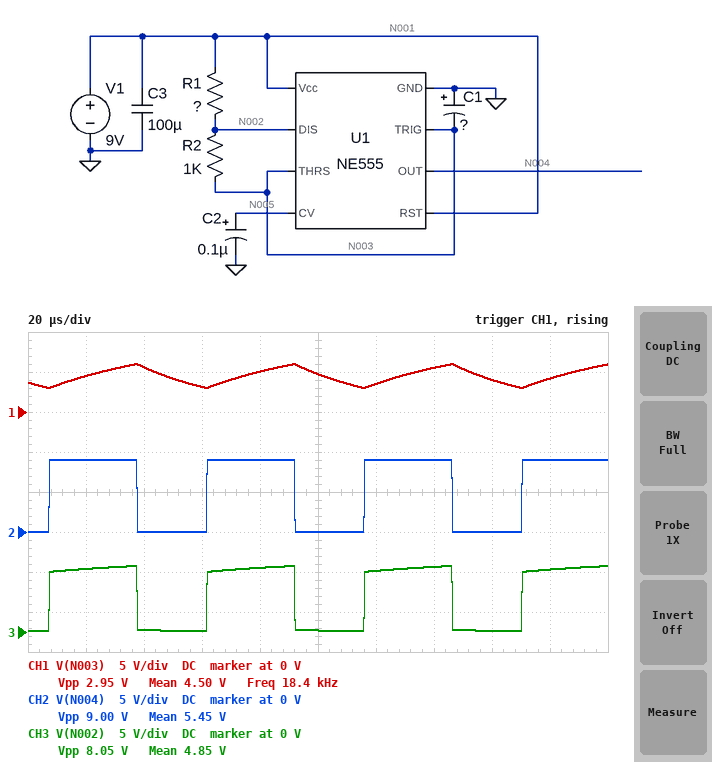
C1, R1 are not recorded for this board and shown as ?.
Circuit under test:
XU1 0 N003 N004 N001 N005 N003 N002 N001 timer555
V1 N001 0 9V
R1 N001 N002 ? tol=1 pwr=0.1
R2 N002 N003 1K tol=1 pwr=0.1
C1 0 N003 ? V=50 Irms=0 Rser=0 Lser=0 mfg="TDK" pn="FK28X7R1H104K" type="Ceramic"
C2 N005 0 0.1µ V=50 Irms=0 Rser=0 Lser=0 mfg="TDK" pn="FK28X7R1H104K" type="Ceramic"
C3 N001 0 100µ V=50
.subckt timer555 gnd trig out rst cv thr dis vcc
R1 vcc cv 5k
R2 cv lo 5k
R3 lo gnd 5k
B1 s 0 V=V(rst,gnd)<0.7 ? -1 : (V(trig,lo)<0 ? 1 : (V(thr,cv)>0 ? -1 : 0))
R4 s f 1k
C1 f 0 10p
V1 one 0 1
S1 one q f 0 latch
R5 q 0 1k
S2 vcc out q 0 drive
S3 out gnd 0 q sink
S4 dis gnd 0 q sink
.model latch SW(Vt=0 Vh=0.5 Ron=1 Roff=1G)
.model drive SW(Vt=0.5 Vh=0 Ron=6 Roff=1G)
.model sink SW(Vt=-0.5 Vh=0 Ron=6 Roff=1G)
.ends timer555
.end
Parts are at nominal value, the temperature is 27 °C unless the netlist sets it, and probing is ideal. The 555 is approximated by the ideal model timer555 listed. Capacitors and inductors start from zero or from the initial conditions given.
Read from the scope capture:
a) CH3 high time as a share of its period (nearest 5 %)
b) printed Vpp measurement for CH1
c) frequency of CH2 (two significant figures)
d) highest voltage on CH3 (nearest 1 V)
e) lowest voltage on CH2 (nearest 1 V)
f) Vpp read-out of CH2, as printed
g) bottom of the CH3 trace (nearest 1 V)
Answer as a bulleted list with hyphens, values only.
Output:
- 55 %
- 2.95 V
- 18 kHz
- 8 V
- 0 V
- 9.00 V
- 0 V
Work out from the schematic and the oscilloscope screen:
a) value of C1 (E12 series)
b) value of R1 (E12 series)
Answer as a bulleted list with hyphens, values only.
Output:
- 33 nF
- 330 Ω
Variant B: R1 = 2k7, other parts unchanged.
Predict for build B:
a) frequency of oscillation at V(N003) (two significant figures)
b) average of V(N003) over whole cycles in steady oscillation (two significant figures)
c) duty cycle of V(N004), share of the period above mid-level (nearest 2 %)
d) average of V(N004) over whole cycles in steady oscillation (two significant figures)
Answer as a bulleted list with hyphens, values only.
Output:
- 9.3 kHz
- 4.6 V
- 78 %
- 7.1 V
